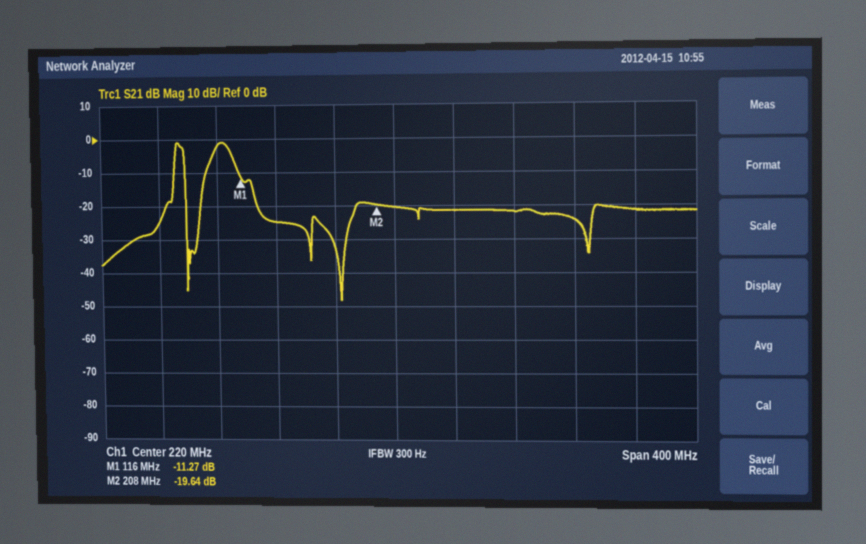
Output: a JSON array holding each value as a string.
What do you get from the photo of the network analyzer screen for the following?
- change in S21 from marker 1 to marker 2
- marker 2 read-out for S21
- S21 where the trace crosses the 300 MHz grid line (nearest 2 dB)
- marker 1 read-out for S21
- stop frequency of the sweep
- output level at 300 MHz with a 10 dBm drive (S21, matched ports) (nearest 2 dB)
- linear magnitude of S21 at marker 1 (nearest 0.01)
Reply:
["-8.37 dB", "-19.64 dB", "-22 dB", "-11.27 dB", "420 MHz", "-12 dBm", "0.27"]
